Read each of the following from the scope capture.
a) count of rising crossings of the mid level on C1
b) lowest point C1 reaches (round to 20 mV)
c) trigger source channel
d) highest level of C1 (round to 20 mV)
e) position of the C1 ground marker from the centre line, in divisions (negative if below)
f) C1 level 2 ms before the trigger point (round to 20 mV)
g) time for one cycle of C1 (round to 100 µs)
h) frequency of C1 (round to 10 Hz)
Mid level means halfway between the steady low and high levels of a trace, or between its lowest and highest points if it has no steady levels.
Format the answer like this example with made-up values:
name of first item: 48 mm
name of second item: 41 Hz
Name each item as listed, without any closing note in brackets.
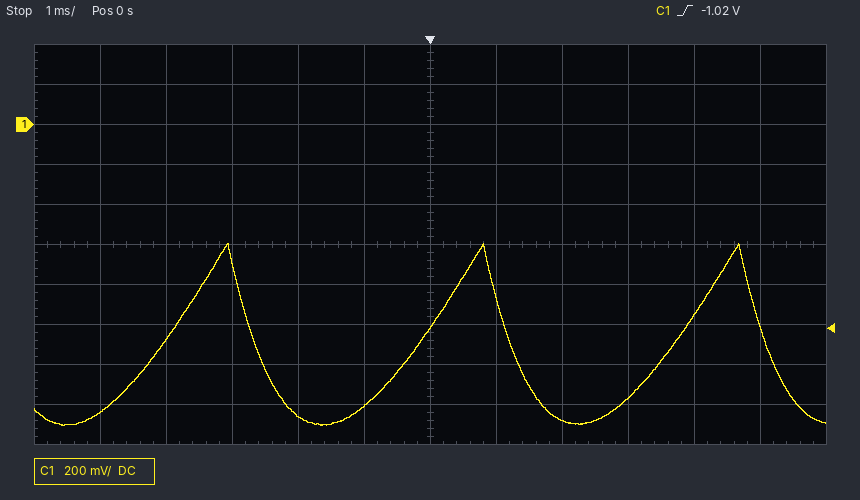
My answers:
count of rising crossings of the mid level on C1: 3
lowest point C1 reaches: -1.50 V
trigger source channel: C1
highest level of C1: -600 mV
position of the C1 ground marker from the centre line, in divisions: +3.0 div
C1 level 2 ms before the trigger point: -1.46 V
time for one cycle of C1: 3.9 ms
frequency of C1: 260 Hz
